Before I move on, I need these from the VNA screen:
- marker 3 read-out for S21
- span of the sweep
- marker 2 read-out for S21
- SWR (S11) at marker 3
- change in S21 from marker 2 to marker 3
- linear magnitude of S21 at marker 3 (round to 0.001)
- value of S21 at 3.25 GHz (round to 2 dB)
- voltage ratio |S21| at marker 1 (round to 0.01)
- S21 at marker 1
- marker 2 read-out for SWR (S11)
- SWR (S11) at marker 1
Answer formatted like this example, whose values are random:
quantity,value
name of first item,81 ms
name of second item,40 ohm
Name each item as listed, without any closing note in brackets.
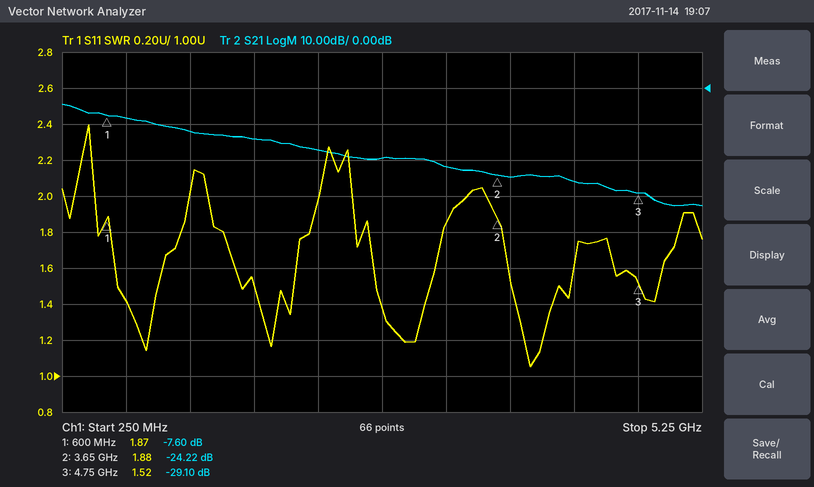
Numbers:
quantity,value
marker 3 read-out for S21,-29.10 dB
span of the sweep,5 GHz
marker 2 read-out for S21,-24.22 dB
SWR (S11) at marker 3,1.52
change in S21 from marker 2 to marker 3,-4.88 dB
linear magnitude of S21 at marker 3,0.035
value of S21 at 3.25 GHz,-22 dB
voltage ratio |S21| at marker 1,0.42
S21 at marker 1,-7.60 dB
marker 2 read-out for SWR,1.88
SWR (S11) at marker 1,1.87
